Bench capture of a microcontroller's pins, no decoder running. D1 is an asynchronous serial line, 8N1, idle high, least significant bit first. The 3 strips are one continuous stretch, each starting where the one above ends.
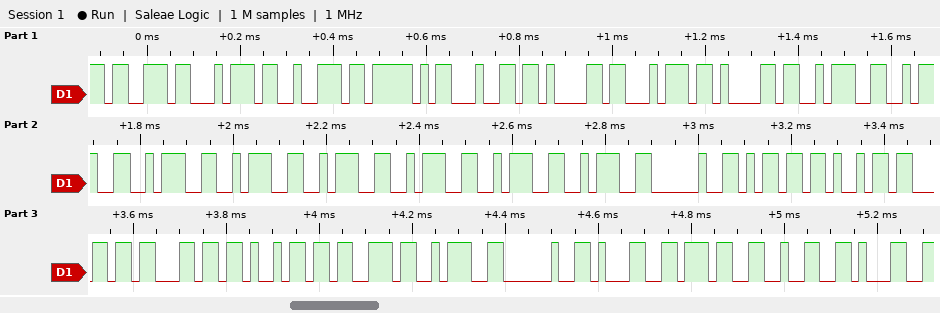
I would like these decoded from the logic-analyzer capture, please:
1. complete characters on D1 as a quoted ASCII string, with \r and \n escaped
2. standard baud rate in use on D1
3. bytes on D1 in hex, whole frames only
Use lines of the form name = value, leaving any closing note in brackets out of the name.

complete characters on D1 as a quoted ASCII string, with \r and \n escaped = "str_data:::::::: millis: 1721"
standard baud rate in use on D1 = 57600 baud
bytes on D1 in hex, whole frames only = 73 74 72 5F 64 61 74 61 3A 3A 3A 3A 3A 3A 3A 3A 20 6D 69 6C 6C 69 73 3A 20 31 37 32 31
